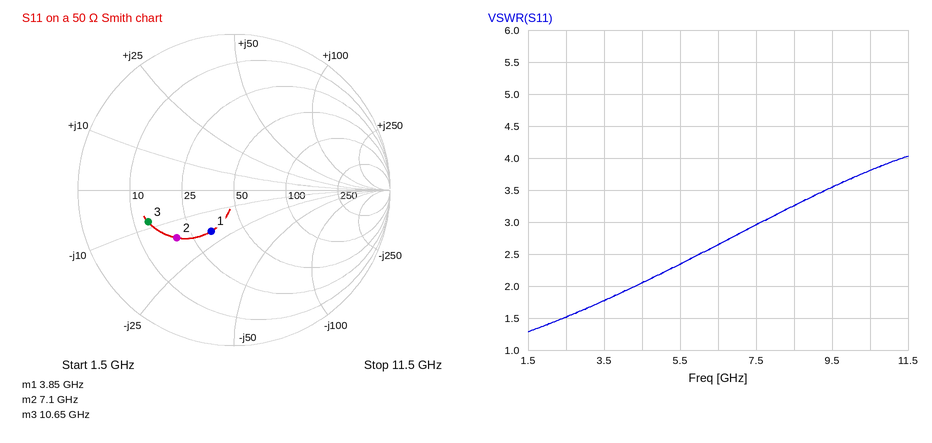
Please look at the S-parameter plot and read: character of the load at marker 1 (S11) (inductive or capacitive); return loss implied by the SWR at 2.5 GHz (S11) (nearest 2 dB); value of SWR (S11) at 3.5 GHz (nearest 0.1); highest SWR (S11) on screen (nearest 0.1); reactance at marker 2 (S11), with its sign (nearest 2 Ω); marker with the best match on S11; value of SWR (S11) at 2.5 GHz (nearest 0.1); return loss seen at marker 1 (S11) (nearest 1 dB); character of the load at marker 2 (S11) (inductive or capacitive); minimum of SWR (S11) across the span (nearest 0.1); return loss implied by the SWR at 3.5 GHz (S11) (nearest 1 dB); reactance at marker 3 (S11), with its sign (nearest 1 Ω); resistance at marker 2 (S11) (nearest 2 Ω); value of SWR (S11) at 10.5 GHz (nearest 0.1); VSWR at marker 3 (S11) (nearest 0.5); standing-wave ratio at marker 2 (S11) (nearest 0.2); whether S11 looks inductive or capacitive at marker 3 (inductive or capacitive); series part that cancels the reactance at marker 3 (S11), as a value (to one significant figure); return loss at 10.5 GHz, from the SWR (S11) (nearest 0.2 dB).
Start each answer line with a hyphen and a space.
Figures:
- capacitive
- 14 dB
- 1.8
- 4.0
- -16 Ω
- marker 1
- 1.5
- 10 dB
- capacitive
- 1.3
- 11 dB
- -8 Ω
- 20 Ω
- 3.8
- 4.0
- 2.8
- capacitive
- 100 pH
- 4.6 dB
